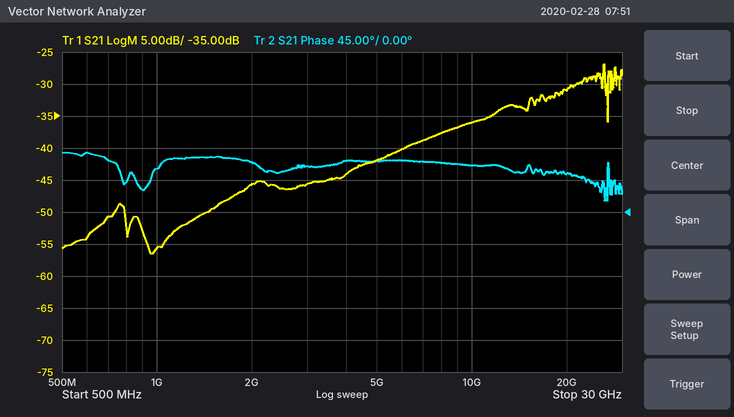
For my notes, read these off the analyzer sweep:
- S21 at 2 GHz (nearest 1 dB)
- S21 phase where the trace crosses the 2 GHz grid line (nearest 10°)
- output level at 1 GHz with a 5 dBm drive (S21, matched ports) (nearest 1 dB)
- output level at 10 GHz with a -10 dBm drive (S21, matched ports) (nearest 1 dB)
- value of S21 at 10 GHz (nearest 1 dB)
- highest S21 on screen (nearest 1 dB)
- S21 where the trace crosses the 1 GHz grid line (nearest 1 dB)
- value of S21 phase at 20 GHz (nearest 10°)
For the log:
-46 dB
70°
-51 dBm
-46 dBm
-36 dB
-27 dB
-56 dB
50°
